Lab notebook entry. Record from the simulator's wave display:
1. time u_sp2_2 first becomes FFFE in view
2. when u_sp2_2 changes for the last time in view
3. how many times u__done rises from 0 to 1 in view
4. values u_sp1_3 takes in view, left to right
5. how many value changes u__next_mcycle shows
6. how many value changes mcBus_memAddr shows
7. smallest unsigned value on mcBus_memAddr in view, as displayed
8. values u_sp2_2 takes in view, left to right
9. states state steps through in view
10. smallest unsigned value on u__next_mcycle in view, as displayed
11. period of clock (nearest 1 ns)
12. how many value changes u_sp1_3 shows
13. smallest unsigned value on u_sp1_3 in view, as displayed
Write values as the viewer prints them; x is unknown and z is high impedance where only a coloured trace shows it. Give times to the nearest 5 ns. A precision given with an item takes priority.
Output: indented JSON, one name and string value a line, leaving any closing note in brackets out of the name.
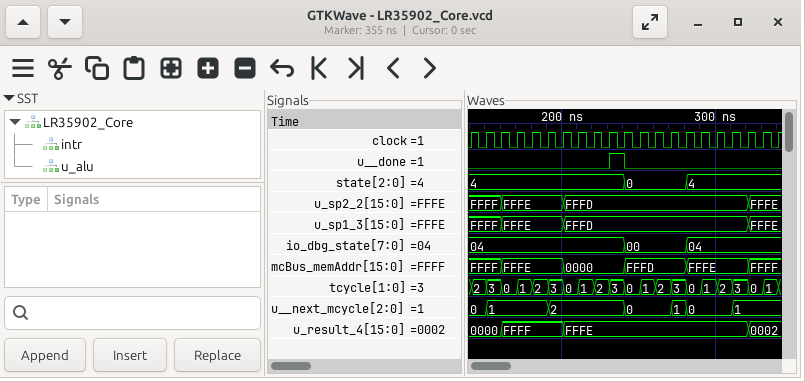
{
  "time u_sp2_2 first becomes FFFE in view": "160 ns",
  "when u_sp2_2 changes for the last time in view": "320 ns",
  "how many times u__done rises from 0 to 1 in view": "1",
  "values u_sp1_3 takes in view, left to right": "FFFF, FFFE, FFFD, FFFE",
  "how many value changes u__next_mcycle shows": "6",
  "how many value changes mcBus_memAddr shows": "5",
  "smallest unsigned value on mcBus_memAddr in view, as displayed": "0000",
  "values u_sp2_2 takes in view, left to right": "FFFF, FFFE, FFFD, FFFE",
  "states state steps through in view": "4, 0, 4",
  "smallest unsigned value on u__next_mcycle in view, as displayed": "0",
  "period of clock": "10 ns",
  "how many value changes u_sp1_3 shows": "3",
  "smallest unsigned value on u_sp1_3 in view, as displayed": "FFFD"
}
